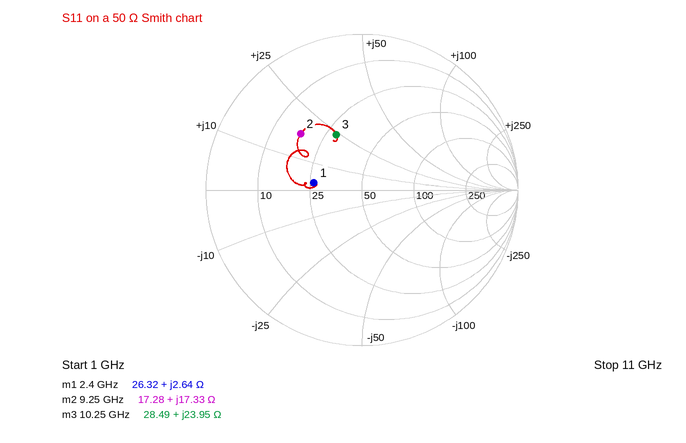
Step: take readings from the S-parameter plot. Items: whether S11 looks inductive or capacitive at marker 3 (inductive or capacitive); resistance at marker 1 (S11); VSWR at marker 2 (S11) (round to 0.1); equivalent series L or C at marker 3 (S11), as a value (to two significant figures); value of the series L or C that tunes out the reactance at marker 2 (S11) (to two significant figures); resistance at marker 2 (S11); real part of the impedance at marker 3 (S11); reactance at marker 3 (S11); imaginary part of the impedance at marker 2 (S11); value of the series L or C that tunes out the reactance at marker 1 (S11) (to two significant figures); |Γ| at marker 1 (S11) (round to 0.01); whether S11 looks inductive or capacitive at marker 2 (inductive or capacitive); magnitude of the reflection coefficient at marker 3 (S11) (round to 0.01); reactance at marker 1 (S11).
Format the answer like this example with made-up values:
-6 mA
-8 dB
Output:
inductive
26.32 Ω
3.3
370 pH
990 fF
17.28 Ω
28.49 Ω
+23.95 Ω
+17.33 Ω
25 pF
0.31
inductive
0.39
+2.64 Ω
